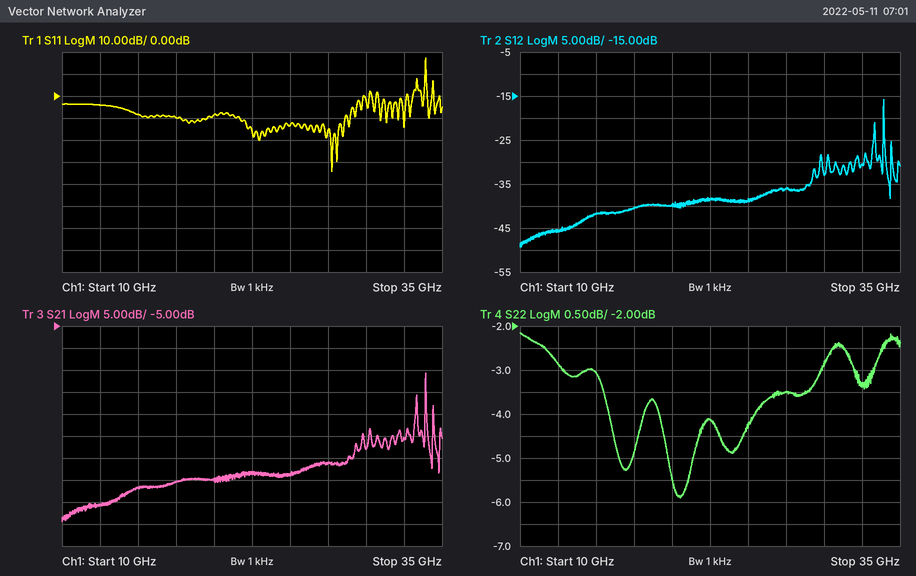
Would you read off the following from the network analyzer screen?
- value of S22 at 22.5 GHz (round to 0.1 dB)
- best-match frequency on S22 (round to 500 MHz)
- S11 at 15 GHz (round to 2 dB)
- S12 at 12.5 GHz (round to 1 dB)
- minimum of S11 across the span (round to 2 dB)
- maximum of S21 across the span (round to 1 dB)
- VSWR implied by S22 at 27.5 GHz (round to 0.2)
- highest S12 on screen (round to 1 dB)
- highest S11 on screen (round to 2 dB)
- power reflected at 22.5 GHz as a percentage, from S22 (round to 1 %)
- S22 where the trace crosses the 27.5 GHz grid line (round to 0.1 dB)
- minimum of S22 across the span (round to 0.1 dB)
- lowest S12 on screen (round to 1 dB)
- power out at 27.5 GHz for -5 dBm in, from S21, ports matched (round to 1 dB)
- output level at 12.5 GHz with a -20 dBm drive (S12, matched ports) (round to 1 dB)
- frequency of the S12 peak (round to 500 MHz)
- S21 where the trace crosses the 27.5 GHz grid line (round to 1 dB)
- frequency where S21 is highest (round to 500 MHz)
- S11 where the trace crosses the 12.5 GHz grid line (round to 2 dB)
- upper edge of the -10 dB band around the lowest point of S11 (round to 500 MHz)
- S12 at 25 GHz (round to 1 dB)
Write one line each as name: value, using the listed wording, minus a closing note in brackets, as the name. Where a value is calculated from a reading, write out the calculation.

value of S22 at 22.5 GHz: -4.1 dB
best-match frequency on S22: 20.5 GHz
S11 at 15 GHz: -8 dB
S12 at 12.5 GHz: -46 dB
minimum of S11 across the span: -34 dB
maximum of S21 across the span: -16 dB
VSWR implied by S22 at 27.5 GHz: |Γ| = 10^(-3.5/20) = 0.6683; VSWR = (1 + 0.6683)/(1 − 0.6683) ≈ 5.0
highest S12 on screen: -16 dB
highest S11 on screen: 18 dB
power reflected at 22.5 GHz as a percentage, from S22: 10^(-4.1/10) ≈ 39 %
S22 where the trace crosses the 27.5 GHz grid line: -3.5 dB
minimum of S22 across the span: -5.9 dB
lowest S12 on screen: -49 dB
power out at 27.5 GHz for -5 dBm in, from S21, ports matched: -5 dBm + (-36 dB) = -41 dBm
output level at 12.5 GHz with a -20 dBm drive (S12, matched ports): -20 dBm + (-46 dB) = -66 dBm
frequency of the S12 peak: 34.0 GHz
S21 where the trace crosses the 27.5 GHz grid line: -36 dB
frequency where S21 is highest: 34.0 GHz
S11 where the trace crosses the 12.5 GHz grid line: -4 dB
upper edge of the -10 dB band around the lowest point of S11: 28.5 GHz
S12 at 25 GHz: -39 dB
